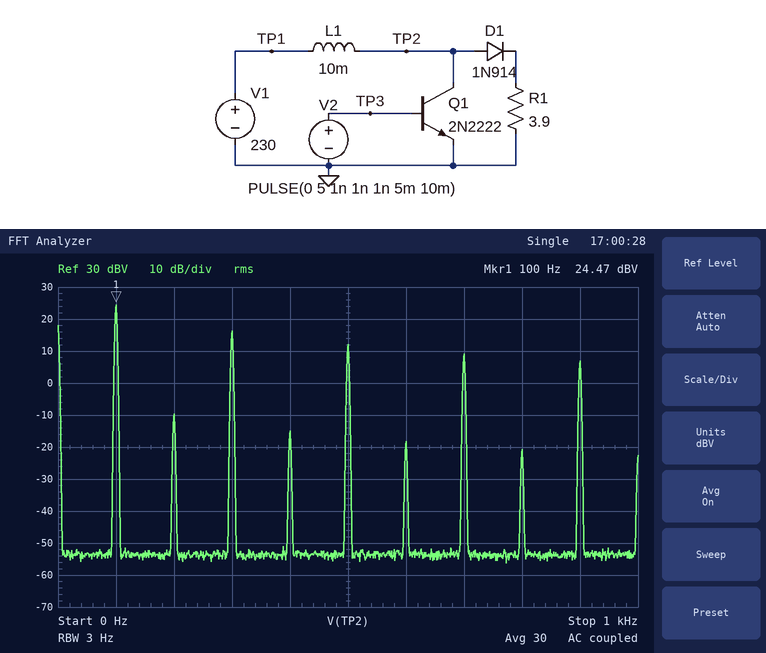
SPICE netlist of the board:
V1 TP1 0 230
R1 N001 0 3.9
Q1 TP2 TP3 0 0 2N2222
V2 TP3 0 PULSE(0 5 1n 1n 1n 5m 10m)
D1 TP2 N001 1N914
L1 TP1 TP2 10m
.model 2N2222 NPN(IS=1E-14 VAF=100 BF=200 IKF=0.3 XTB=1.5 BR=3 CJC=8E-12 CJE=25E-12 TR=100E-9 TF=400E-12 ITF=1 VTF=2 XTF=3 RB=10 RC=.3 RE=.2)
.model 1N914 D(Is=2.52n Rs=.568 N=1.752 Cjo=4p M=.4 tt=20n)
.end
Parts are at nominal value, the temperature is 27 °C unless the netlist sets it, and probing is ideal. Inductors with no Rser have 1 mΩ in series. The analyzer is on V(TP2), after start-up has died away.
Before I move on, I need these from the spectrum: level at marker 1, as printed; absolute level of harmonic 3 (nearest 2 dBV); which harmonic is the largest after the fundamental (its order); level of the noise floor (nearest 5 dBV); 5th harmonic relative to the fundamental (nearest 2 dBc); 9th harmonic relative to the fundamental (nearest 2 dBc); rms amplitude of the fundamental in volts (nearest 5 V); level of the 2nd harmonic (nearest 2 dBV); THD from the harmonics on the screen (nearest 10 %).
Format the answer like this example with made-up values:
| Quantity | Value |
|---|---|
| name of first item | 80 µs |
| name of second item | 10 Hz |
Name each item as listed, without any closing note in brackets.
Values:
| Quantity | Value |
|---|---|
| level at marker 1, as printed | 24.47 dBV |
| absolute level of harmonic 3 | 16 dBV |
| which harmonic is the largest after the fundamental | 3 |
| level of the noise floor | -55 dBV |
| 5th harmonic relative to the fundamental | -12 dBc |
| 9th harmonic relative to the fundamental | -18 dBc |
| rms amplitude of the fundamental in volts | 15 V |
| level of the 2nd harmonic | -10 dBV |
| THD from the harmonics on the screen | 50 % |
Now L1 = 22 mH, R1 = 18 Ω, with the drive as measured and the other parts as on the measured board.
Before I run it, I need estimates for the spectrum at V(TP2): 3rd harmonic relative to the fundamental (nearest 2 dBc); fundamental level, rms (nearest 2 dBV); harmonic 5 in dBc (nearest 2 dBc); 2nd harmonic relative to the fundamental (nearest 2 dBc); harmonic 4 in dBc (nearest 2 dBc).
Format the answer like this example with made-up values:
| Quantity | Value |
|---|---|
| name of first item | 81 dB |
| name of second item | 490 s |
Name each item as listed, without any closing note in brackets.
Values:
| Quantity | Value |
|---|---|
| 3rd harmonic relative to the fundamental | -6 dBc |
| fundamental level, rms | 34 dBV |
| harmonic 5 in dBc | -10 dBc |
| 2nd harmonic relative to the fundamental | -20 dBc |
| harmonic 4 in dBc | -24 dBc |
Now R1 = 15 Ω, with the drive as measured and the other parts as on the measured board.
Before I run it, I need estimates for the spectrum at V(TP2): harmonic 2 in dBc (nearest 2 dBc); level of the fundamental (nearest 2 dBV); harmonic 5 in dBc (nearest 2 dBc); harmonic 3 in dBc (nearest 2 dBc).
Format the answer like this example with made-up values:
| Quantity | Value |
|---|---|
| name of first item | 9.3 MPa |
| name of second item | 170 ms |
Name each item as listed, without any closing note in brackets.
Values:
| Quantity | Value |
|---|---|
| harmonic 2 in dBc | -22 dBc |
| level of the fundamental | 28 dBV |
| harmonic 5 in dBc | -8 dBc |
| harmonic 3 in dBc | -4 dBc |
